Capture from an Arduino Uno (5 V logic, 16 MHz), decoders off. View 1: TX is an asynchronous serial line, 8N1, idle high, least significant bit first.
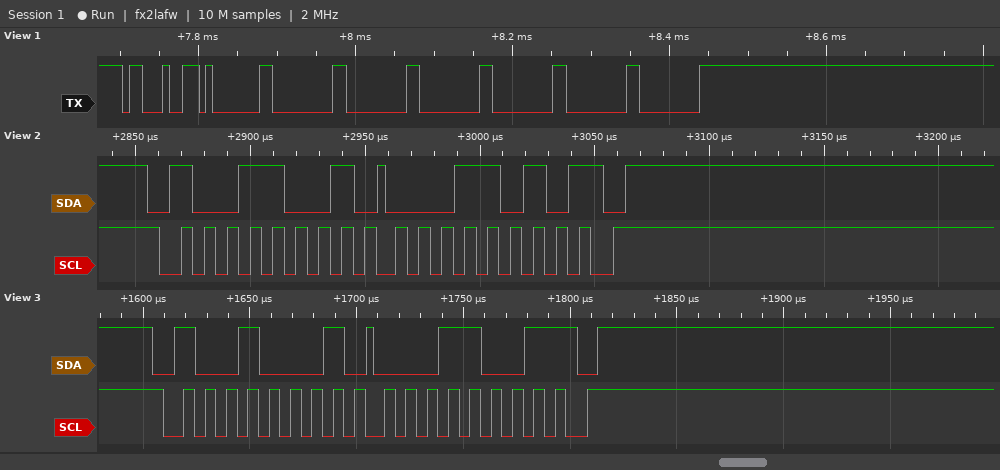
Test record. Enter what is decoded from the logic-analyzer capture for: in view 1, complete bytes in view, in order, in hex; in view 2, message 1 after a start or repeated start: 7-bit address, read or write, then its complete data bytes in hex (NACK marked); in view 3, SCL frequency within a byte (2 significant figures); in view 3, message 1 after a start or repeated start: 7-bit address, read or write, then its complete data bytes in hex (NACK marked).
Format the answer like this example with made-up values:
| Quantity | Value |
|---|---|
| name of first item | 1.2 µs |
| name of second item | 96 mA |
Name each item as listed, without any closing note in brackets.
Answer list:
| Quantity | Value |
|---|---|
| in view 1, complete bytes in view, in order, in hex | 23 01 00 00 00 00 00 00 |
| in view 2, message 1 after a start or repeated start: 7-bit address, read or write, then its complete data bytes in hex | 0x4C read: 1A NACK |
| in view 3, SCL frequency within a byte | 100 kHz |
| in view 3, message 1 after a start or repeated start: 7-bit address, read or write, then its complete data bytes in hex | 0x48 read: 19 NACK |
